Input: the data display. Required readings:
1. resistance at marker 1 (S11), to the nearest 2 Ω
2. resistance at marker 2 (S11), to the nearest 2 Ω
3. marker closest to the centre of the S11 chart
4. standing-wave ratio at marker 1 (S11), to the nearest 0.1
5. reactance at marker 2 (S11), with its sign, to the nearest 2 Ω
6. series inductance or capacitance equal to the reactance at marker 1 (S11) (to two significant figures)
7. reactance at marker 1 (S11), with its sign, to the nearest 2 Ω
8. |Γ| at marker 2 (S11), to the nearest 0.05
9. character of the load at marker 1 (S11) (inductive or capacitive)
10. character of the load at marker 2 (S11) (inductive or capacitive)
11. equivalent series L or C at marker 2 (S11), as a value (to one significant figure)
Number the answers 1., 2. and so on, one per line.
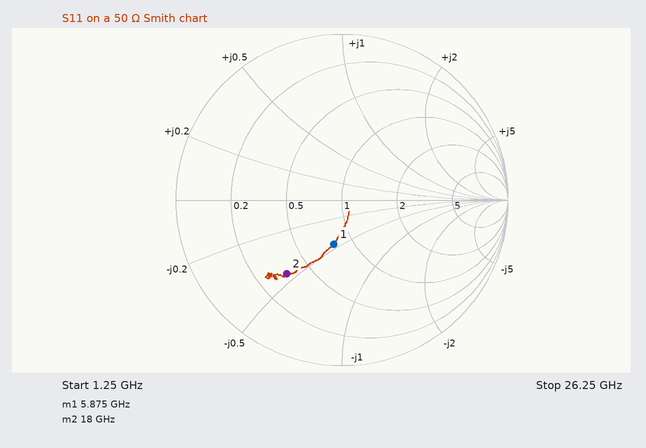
1. 40 Ω
2. 18 Ω
3. marker 1
4. 1.7
5. -22 Ω
6. 1.2 pF
7. -22 Ω
8. 0.55
9. capacitive
10. capacitive
11. 400 fF
